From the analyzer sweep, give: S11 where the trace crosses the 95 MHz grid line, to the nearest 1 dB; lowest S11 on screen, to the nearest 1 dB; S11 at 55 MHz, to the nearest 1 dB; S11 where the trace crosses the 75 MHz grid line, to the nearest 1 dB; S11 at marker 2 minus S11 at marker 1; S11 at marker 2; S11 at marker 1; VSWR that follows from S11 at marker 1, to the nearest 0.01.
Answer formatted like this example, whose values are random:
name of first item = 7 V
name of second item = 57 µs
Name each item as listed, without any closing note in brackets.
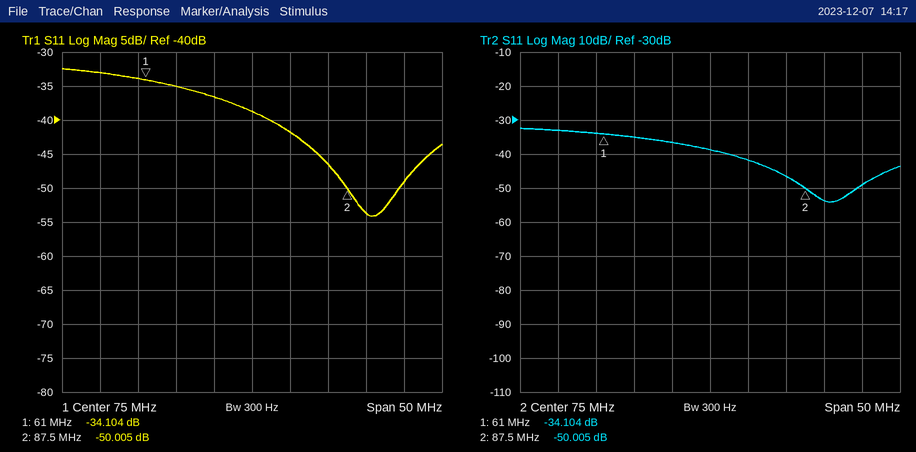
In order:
S11 where the trace crosses the 95 MHz grid line, to the nearest 1 dB = -49 dB
lowest S11 on screen, to the nearest 1 dB = -54 dB
S11 at 55 MHz, to the nearest 1 dB = -33 dB
S11 where the trace crosses the 75 MHz grid line, to the nearest 1 dB = -39 dB
S11 at marker 2 minus S11 at marker 1 = -15.901 dB
S11 at marker 2 = -50.005 dB
S11 at marker 1 = -34.104 dB
VSWR that follows from S11 at marker 1, to the nearest 0.01 = 1.04
